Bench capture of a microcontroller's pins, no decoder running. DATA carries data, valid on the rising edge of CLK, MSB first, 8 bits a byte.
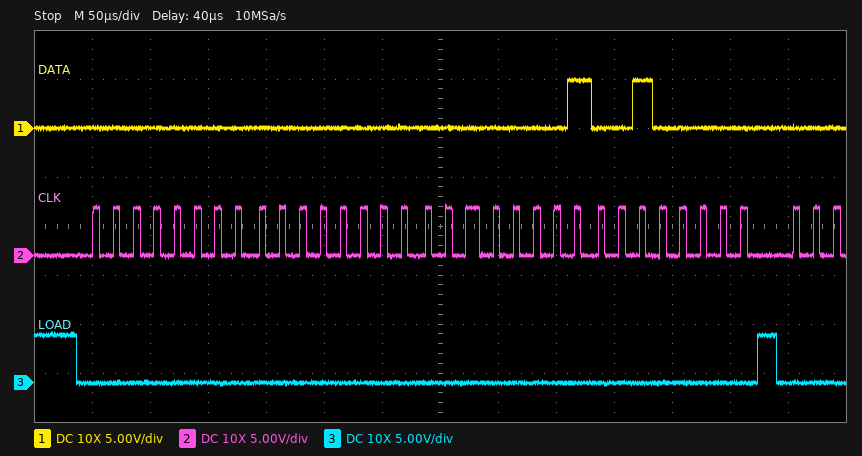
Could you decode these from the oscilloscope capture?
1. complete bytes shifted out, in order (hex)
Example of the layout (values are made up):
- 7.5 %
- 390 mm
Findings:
- 0x00 0x00 0x01 0x20
